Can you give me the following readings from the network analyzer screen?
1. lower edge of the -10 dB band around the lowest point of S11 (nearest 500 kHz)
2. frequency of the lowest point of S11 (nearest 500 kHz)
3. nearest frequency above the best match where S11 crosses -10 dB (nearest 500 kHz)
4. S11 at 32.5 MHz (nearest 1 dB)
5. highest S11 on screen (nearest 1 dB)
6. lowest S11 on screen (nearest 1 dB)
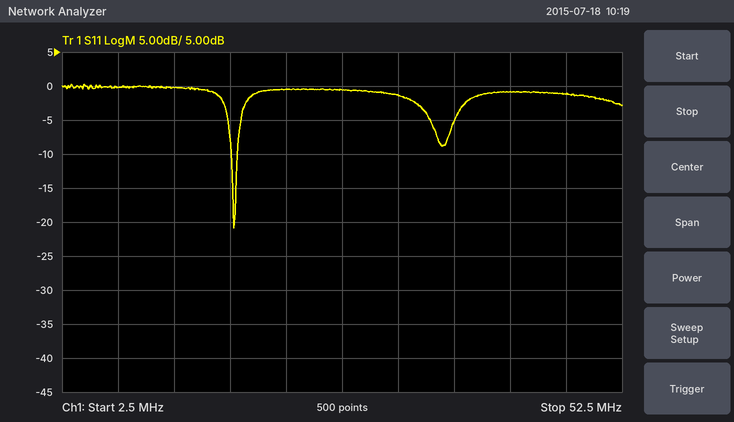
17.5 MHz
18.0 MHz
18.0 MHz
-1 dB
0 dB
-21 dB
